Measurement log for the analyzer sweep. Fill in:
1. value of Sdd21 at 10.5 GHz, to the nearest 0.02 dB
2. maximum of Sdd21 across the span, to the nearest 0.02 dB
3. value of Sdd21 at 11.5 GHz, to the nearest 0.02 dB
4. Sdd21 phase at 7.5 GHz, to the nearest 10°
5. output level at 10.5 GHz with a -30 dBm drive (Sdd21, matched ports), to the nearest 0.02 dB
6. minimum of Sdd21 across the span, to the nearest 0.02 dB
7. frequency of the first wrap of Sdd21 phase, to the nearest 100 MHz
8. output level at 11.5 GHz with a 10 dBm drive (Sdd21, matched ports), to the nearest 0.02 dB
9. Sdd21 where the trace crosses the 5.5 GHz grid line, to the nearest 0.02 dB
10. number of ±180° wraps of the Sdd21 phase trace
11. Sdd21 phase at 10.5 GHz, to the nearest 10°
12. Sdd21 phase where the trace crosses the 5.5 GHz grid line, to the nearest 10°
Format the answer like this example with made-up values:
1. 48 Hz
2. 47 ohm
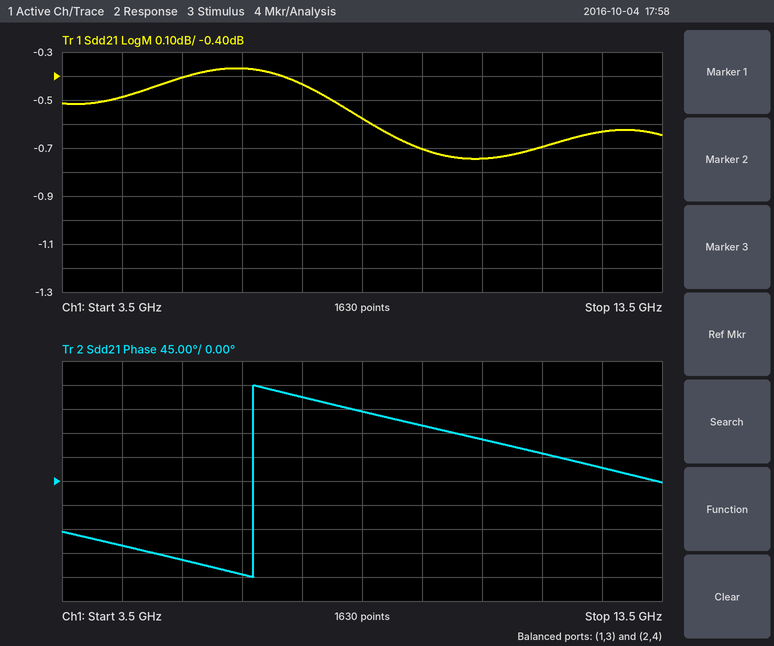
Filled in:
1. -0.74 dB
2. -0.36 dB
3. -0.70 dB
4. 160°
5. -30.74 dBm
6. -0.74 dB
7. 6.7 GHz
8. 9.30 dBm
9. -0.40 dB
10. 1
11. 80°
12. -150°
